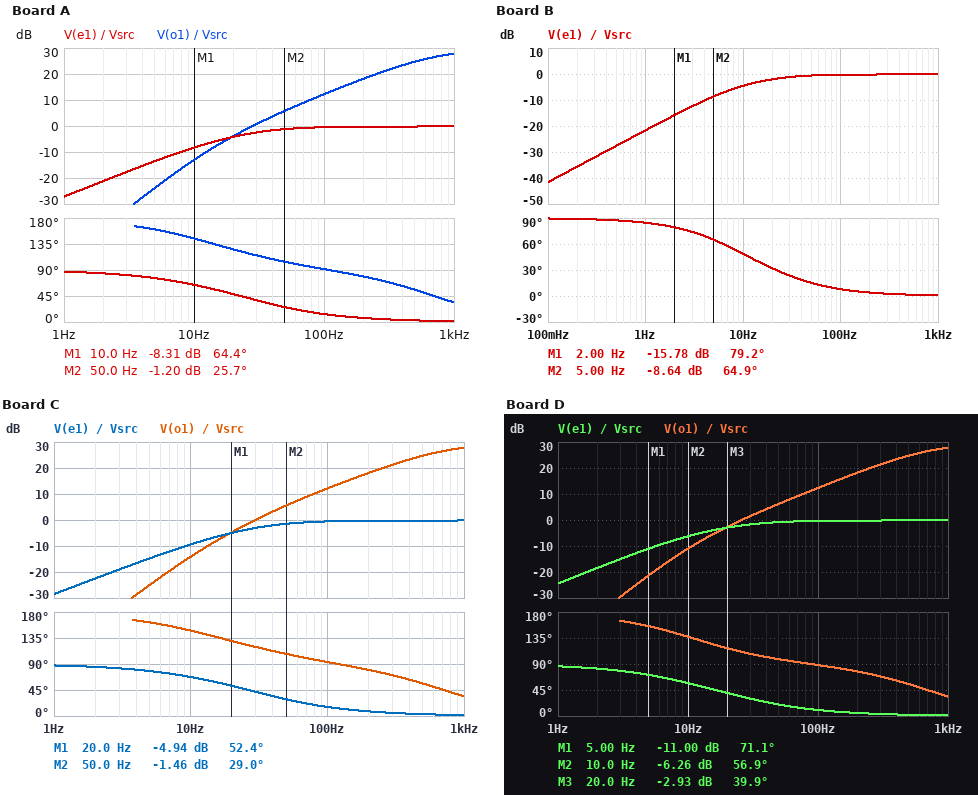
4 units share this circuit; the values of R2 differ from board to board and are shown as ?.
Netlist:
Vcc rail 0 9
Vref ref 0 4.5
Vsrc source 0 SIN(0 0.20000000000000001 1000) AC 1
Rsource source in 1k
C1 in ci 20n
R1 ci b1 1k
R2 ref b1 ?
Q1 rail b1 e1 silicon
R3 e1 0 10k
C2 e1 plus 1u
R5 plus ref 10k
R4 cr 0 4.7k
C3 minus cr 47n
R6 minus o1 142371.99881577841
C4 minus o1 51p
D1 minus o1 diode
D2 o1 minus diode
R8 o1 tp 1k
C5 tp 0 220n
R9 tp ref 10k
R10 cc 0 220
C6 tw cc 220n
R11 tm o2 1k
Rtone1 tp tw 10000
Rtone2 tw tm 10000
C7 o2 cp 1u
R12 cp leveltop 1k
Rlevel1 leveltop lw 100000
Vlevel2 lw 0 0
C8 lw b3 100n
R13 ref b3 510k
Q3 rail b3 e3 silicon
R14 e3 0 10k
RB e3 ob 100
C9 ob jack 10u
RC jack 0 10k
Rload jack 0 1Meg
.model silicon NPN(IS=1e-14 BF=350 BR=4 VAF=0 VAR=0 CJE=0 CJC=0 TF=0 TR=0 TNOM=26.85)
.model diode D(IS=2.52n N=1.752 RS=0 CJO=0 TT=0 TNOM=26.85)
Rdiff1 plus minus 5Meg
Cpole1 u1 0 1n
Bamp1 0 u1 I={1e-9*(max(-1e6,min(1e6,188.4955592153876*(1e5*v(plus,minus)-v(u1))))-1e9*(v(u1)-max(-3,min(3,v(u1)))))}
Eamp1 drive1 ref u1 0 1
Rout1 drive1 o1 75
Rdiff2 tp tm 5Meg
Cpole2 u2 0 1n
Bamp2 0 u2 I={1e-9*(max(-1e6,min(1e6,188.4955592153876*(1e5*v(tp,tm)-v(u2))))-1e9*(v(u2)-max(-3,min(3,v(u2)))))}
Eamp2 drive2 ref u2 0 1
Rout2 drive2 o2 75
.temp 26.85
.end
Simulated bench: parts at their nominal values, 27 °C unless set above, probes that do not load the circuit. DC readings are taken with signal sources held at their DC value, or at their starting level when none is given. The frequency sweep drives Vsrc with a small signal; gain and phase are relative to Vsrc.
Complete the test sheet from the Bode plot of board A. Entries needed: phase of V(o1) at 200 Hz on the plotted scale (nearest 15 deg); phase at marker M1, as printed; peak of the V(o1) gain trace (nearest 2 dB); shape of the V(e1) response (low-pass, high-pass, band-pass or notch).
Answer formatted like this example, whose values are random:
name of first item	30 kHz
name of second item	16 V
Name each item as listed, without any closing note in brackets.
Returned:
phase of V(o1) at 200 Hz on the plotted scale	75 deg
phase at marker M1, as printed	64.4 deg
peak of the V(o1) gain trace	28 dB
shape of the V(e1) response	high-pass
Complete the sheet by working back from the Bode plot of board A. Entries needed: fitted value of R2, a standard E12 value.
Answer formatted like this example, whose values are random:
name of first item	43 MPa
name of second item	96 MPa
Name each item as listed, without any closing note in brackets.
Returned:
fitted value of R2, a standard E12 value	390 kΩ
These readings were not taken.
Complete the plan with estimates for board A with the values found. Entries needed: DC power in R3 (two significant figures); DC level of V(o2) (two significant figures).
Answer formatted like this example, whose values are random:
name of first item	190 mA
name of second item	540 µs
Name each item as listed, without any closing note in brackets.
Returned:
DC power in R3	1.2 mW
DC level of V(o2)	4.5 V
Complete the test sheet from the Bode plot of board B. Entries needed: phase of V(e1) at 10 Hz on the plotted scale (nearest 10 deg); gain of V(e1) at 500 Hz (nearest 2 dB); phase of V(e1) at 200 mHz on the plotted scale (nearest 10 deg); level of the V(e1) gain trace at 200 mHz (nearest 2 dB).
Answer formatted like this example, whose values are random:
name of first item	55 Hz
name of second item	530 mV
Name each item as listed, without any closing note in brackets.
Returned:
phase of V(e1) at 10 Hz on the plotted scale	50 deg
gain of V(e1) at 500 Hz	0 dB
phase of V(e1) at 200 mHz on the plotted scale	90 deg
level of the V(e1) gain trace at 200 mHz	-36 dB
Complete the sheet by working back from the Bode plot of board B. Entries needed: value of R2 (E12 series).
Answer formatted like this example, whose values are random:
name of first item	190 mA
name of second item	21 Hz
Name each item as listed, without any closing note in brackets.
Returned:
value of R2	820 kΩ
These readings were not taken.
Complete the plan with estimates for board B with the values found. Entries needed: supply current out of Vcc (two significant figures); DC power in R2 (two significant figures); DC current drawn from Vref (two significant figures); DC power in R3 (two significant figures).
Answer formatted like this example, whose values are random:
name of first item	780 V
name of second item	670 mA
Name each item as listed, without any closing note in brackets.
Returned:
supply current out of Vcc	650 µA
DC power in R2	660 nW
DC current drawn from Vref	1.9 µA
DC power in R3	990 µW
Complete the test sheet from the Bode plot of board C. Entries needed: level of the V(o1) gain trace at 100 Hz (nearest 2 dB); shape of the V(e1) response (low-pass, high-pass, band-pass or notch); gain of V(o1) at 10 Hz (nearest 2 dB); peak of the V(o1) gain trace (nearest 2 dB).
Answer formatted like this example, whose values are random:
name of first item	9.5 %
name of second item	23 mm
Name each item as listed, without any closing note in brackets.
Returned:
level of the V(o1) gain trace at 100 Hz	12 dB
shape of the V(e1) response	high-pass
gain of V(o1) at 10 Hz	-14 dB
peak of the V(o1) gain trace	28 dB
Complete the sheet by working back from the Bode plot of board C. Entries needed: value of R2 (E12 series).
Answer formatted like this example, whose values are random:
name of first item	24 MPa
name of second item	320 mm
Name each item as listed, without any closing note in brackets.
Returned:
value of R2	330 kΩ
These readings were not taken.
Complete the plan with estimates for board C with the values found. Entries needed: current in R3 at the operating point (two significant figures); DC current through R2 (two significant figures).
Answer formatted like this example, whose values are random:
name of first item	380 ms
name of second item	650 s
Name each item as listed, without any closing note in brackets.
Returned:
current in R3 at the operating point	350 µA
DC current through R2	1.0 µA
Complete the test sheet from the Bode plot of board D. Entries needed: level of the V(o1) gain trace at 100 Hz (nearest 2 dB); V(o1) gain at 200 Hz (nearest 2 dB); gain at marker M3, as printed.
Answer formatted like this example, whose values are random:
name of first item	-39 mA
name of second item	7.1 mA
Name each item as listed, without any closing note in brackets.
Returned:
level of the V(o1) gain trace at 100 Hz	12 dB
V(o1) gain at 200 Hz	18 dB
gain at marker M3, as printed	-2.93 dB
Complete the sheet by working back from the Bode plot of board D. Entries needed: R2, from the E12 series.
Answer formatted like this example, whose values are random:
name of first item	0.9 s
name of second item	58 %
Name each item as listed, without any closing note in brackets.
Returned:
R2, from the E12 series	560 kΩ
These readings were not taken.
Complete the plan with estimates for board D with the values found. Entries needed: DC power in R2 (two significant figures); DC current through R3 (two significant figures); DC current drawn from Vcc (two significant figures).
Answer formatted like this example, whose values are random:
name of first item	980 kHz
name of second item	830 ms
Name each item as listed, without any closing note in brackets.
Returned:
DC power in R2	510 nW
DC current through R3	330 µA
DC current drawn from Vcc	670 µA
